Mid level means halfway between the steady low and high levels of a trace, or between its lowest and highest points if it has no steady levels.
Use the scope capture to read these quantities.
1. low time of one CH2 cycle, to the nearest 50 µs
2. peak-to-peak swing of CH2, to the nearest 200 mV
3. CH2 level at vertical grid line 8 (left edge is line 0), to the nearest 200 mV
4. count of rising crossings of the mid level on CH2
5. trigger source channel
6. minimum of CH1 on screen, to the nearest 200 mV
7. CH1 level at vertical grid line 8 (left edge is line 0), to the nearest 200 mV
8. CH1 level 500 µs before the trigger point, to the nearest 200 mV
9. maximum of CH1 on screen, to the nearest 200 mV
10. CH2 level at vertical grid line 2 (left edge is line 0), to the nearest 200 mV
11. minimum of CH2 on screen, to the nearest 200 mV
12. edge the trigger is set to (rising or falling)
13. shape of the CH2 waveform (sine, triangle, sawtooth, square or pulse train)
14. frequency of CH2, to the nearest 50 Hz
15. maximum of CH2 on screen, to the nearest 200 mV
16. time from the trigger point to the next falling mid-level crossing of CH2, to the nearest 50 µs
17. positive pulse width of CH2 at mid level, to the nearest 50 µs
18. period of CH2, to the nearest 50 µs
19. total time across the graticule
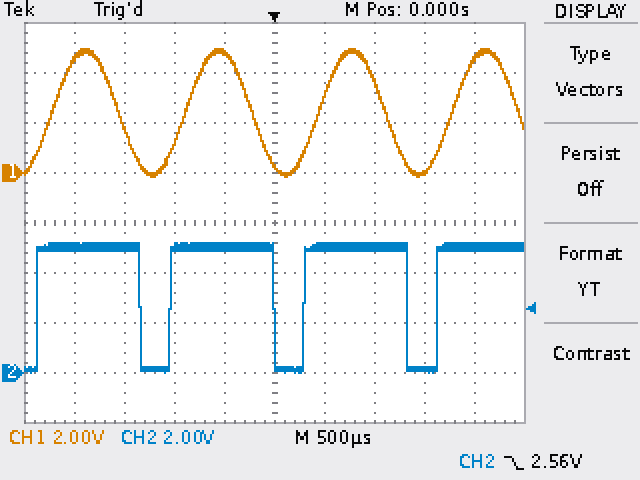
300 µs
5.2 V
200 mV
4
CH2
-200 mV
0.0 V
4.8 V
5.0 V
5.0 V
0.0 V
falling
pulse train
750 Hz
5.2 V
1.35 ms
1.05 ms
1.35 ms
5 ms
